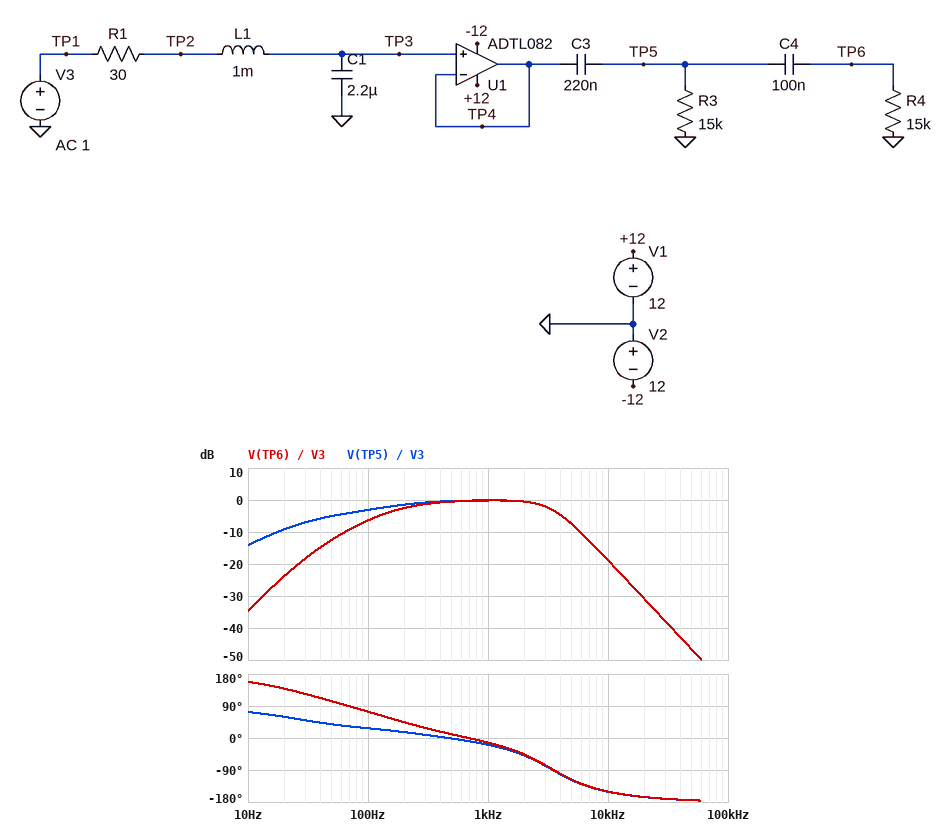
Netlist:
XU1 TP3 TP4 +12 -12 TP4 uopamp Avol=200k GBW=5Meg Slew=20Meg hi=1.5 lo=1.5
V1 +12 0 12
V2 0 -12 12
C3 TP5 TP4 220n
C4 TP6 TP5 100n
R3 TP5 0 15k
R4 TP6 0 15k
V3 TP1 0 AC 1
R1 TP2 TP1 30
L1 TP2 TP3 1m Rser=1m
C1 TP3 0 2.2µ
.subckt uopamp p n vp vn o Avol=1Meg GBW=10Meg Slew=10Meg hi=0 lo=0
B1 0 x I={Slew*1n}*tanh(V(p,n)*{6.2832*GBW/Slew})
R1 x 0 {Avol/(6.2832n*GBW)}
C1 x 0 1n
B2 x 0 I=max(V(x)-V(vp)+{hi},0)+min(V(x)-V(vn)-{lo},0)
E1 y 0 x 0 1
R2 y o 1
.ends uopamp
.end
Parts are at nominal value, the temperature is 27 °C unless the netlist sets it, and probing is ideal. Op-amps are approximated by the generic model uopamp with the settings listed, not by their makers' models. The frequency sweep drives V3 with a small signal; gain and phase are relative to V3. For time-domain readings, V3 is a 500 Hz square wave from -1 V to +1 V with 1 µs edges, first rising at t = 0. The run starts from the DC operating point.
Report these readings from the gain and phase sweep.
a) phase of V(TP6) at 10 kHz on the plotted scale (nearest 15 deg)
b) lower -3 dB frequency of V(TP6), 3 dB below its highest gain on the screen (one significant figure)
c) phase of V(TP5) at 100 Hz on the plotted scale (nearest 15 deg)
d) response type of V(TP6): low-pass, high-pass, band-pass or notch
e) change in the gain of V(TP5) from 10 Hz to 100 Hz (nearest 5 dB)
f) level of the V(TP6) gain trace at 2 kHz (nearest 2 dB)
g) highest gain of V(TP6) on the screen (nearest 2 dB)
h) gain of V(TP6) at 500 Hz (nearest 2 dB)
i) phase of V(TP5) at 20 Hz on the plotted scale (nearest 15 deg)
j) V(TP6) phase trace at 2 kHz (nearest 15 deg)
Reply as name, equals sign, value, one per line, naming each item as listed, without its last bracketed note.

phase of V(TP6) at 10 kHz on the plotted scale = -150 deg
lower -3 dB frequency of V(TP6), 3 dB below its highest gain on the screen = 200 Hz
phase of V(TP5) at 100 Hz on the plotted scale = 30 deg
response type of V(TP6): low-pass, high-pass, band-pass or notch = band-pass
change in the gain of V(TP5) from 10 Hz to 100 Hz = 10 dB
level of the V(TP6) gain trace at 2 kHz = 0 dB
highest gain of V(TP6) on the screen = 0 dB
gain of V(TP6) at 500 Hz = 0 dB
phase of V(TP5) at 20 Hz on the plotted scale = 60 deg
V(TP6) phase trace at 2 kHz = -45 deg
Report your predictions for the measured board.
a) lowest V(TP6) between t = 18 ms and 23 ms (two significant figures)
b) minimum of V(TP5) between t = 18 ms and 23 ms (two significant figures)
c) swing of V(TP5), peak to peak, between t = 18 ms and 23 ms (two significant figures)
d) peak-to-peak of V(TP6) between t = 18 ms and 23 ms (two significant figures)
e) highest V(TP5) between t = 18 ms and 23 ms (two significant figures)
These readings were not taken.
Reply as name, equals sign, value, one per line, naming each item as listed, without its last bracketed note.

lowest V(TP6) between t = 18 ms and 23 ms = -1.5 V
minimum of V(TP5) between t = 18 ms and 23 ms = -1.3 V
swing of V(TP5), peak to peak, between t = 18 ms and 23 ms = 2.5 V
peak-to-peak of V(TP6) between t = 18 ms and 23 ms = 2.9 V
highest V(TP5) between t = 18 ms and 23 ms = 1.3 V
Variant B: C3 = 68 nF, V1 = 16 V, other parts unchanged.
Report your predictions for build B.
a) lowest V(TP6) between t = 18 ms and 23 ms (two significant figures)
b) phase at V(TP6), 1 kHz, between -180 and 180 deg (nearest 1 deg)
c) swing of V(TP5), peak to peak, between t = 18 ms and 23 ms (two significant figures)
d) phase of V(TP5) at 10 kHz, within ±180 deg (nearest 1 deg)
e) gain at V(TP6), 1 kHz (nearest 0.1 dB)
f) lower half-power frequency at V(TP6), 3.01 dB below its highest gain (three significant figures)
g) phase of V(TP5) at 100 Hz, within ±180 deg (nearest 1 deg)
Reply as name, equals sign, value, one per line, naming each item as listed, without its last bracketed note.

lowest V(TP6) between t = 18 ms and 23 ms = -1.6 V
phase at V(TP6), 1 kHz, between -180 and 180 deg = -1 deg
swing of V(TP5), peak to peak, between t = 18 ms and 23 ms = 2.9 V
phase of V(TP5) at 10 kHz, within ±180 deg = -150 deg
gain at V(TP6), 1 kHz = -0.6 dB
lower half-power frequency at V(TP6), 3.01 dB below its highest gain = 347 Hz
phase of V(TP5) at 100 Hz, within ±180 deg = 50 deg
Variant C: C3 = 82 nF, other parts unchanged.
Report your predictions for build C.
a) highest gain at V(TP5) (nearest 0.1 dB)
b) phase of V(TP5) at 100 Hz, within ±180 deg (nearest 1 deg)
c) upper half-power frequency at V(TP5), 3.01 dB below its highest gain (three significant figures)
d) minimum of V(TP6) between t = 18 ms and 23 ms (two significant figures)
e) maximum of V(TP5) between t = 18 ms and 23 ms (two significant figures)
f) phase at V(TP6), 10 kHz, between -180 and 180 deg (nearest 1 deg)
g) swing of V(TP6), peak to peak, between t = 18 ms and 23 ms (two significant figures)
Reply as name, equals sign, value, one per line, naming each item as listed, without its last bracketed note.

highest gain at V(TP5) = -0.3 dB
phase of V(TP5) at 100 Hz, within ±180 deg = 47 deg
upper half-power frequency at V(TP5), 3.01 dB below its highest gain = 3.52 kHz
minimum of V(TP6) between t = 18 ms and 23 ms = -1.6 V
maximum of V(TP5) between t = 18 ms and 23 ms = 1.4 V
phase at V(TP6), 10 kHz, between -180 and 180 deg = -150 deg
swing of V(TP6), peak to peak, between t = 18 ms and 23 ms = 3.1 V
